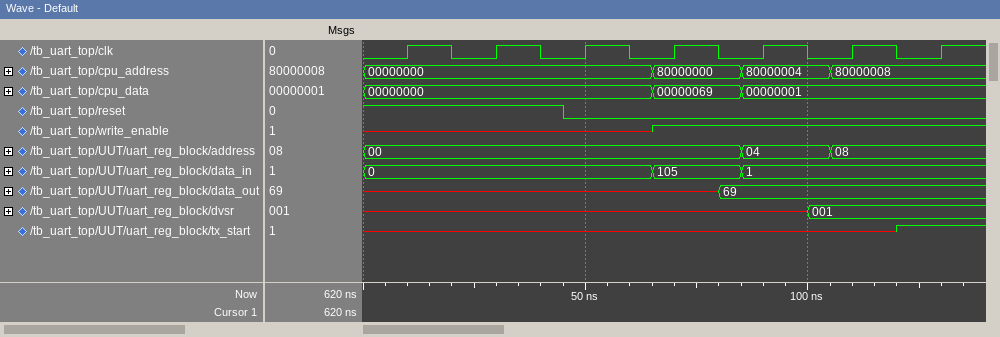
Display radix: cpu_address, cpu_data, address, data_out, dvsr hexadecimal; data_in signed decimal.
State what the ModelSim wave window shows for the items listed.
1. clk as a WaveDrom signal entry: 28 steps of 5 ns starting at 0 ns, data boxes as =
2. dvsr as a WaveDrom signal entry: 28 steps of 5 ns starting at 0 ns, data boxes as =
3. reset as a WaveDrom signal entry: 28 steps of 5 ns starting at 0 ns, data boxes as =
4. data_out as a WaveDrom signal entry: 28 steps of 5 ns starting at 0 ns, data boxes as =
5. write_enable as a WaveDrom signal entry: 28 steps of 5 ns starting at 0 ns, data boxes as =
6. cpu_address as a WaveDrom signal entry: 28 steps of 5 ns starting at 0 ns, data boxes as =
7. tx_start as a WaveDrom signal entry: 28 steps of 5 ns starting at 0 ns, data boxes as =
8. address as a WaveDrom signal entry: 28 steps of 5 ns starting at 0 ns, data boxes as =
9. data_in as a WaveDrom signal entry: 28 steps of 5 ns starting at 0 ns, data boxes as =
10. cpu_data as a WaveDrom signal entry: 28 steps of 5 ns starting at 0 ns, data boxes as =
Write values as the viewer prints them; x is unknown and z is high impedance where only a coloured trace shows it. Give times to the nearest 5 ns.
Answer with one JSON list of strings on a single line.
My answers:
["{name: 'clk', wave: '0.1.0.1.0.1.0.1.0.1.0.1.0.1.'}", "{name: 'dvsr', wave: 'x...................=.......', data: '001'}", "{name: 'reset', wave: '1........0..................'}", "{name: 'data_out', wave: 'x...............=...........', data: '69'}", "{name: 'write_enable', wave: 'x............1..............'}", "{name: 'cpu_address', wave: '=............=...=...=......', data: '00000000 80000000 80000004 80000008'}", "{name: 'tx_start', wave: 'x.......................1...'}", "{name: 'address', wave: '=................=...=......', data: '00 04 08'}", "{name: 'data_in', wave: '=............=...=..........', data: '0 105 1'}", "{name: 'cpu_data', wave: '=............=...=..........', data: '00000000 00000069 00000001'}"]
